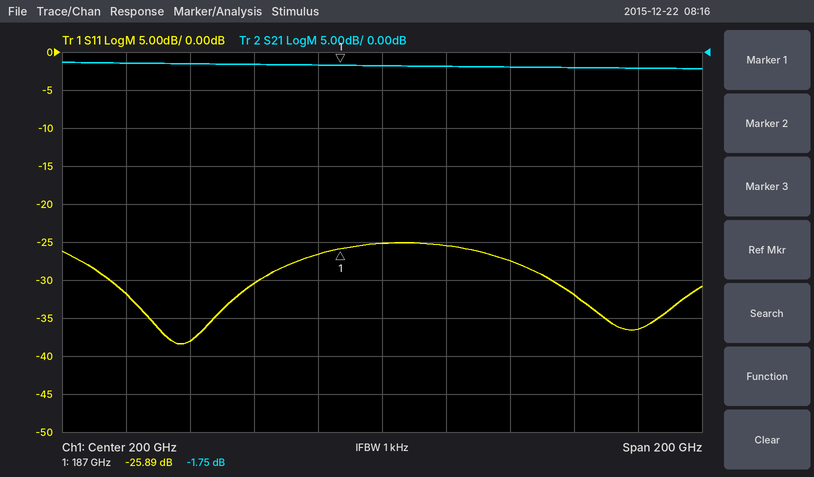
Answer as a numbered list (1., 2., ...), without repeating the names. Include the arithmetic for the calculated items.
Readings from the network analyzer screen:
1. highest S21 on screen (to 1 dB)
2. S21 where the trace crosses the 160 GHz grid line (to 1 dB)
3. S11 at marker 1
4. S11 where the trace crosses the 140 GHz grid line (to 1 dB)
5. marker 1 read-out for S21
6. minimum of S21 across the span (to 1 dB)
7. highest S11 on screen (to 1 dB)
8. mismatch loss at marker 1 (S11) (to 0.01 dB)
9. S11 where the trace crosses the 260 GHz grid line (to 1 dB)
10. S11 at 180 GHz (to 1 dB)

1. -1 dB
2. -2 dB
3. -25.89 dB
4. -38 dB
5. -1.75 dB
6. -2 dB
7. -25 dB
8. −10 log10(1 − 10^(-25.89/10)) ≈ 0.01 dB
9. -32 dB
10. -27 dB
